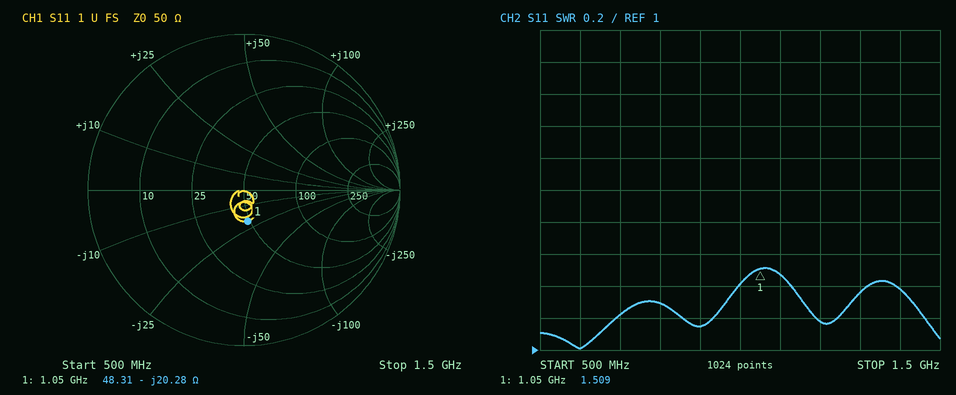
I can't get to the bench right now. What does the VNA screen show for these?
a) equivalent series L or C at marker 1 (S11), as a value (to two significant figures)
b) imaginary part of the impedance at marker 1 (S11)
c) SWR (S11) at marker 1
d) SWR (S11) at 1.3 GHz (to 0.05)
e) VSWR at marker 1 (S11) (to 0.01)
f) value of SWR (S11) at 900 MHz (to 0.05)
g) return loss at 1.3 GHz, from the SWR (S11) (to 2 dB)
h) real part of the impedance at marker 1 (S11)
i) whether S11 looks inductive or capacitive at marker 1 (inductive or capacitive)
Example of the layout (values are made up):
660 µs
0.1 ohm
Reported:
7.5 pF
-20.28 Ω
1.509
1.35
1.51
1.15
16 dB
48.31 Ω
capacitive
